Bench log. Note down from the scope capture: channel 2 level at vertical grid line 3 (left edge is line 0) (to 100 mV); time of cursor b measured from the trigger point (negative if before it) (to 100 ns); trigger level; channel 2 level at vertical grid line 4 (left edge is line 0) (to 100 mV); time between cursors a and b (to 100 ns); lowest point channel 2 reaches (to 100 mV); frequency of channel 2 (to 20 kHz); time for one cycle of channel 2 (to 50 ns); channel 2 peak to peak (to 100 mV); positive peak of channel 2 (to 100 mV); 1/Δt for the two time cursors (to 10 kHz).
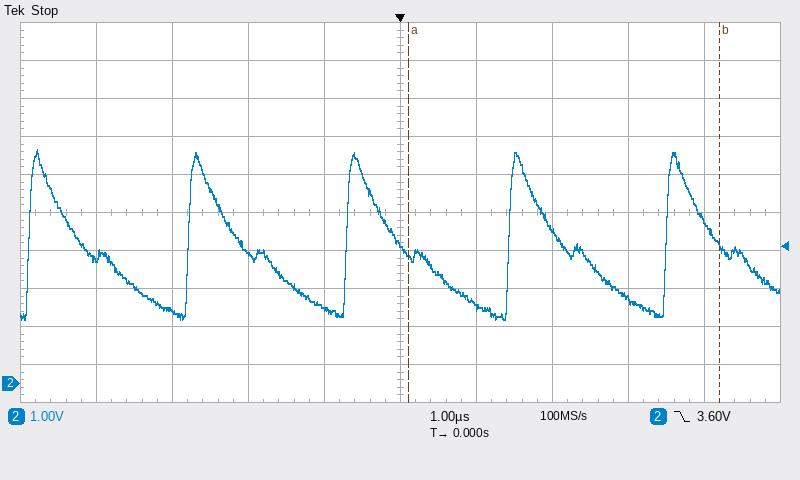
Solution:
3.4 V
+4.2 µs
3.60 V
2.0 V
4.1 µs
1.7 V
480 kHz
2.10 µs
4.5 V
6.2 V
240 kHz
